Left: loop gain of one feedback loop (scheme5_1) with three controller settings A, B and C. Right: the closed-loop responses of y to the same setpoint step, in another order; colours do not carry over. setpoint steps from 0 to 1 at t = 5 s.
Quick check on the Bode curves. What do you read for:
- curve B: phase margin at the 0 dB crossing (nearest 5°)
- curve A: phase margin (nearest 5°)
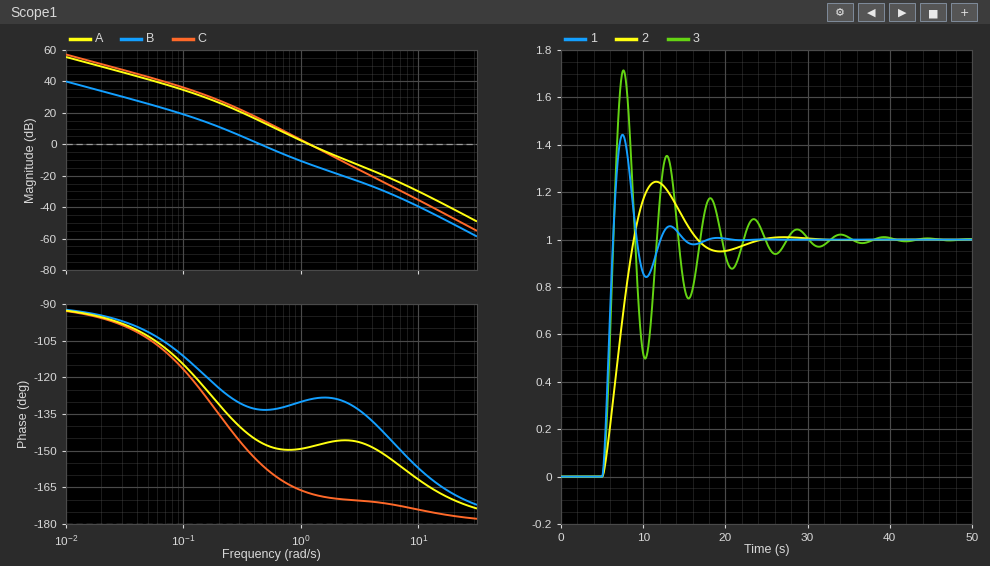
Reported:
45°
30°
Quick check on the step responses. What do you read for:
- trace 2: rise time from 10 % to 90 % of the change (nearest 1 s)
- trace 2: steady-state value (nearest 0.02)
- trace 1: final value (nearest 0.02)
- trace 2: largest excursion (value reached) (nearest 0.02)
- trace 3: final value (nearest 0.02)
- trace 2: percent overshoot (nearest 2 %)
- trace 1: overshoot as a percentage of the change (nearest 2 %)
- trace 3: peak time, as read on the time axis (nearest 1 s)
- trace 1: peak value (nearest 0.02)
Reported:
3 s
1.00
1.00
1.24
1.00
24 %
44 %
8 s
1.44
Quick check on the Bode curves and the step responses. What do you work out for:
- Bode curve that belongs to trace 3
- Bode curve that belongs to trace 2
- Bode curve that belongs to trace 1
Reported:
C
B
A
